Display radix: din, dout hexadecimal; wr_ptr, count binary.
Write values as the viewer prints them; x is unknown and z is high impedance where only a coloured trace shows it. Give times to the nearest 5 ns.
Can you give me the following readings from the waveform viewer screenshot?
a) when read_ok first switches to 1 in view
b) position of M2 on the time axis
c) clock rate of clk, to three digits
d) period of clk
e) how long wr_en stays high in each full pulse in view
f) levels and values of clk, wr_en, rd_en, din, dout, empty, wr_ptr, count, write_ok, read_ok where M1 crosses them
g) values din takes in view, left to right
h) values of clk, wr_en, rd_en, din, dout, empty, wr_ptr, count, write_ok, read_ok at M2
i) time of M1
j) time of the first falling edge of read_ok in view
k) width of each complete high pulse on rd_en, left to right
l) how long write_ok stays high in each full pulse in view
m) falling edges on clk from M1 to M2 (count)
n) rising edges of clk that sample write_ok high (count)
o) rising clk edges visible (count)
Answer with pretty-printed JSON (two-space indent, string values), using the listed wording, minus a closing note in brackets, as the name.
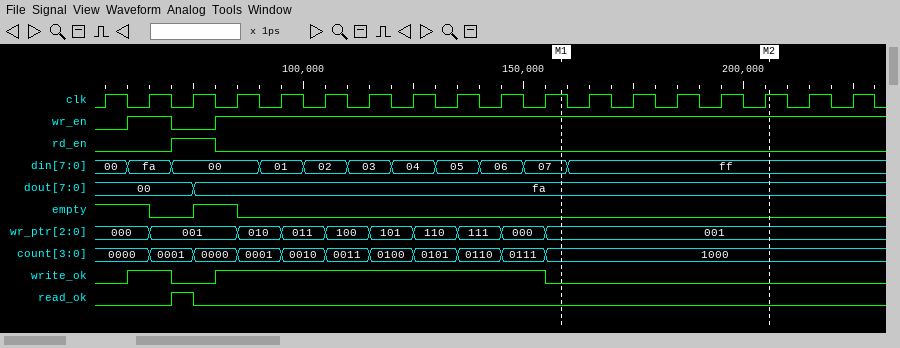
{
  "when read_ok first switches to 1 in view": "70 ns",
  "position of M2 on the time axis": "205 ns",
  "clock rate of clk, to three digits": "100 MHz",
  "period of clk": "10 ns",
  "how long wr_en stays high in each full pulse in view": "10 ns",
  "levels and values of clk, wr_en, rd_en, din, dout, empty, wr_ptr, count, write_ok, read_ok where M1 crosses them": "clk=1, wr_en=1, rd_en=0, din=07, dout=fa, empty=0, wr_ptr=001, count=1000, write_ok=0, read_ok=0",
  "values din takes in view, left to right": "00, fa, 00, 01, 02, 03, 04, 05, 06, 07, ff",
  "values of clk, wr_en, rd_en, din, dout, empty, wr_ptr, count, write_ok, read_ok at M2": "clk=1, wr_en=1, rd_en=0, din=ff, dout=fa, empty=0, wr_ptr=001, count=1000, write_ok=0, read_ok=0",
  "time of M1": "160 ns",
  "time of the first falling edge of read_ok in view": "75 ns",
  "width of each complete high pulse on rd_en, left to right": "10 ns",
  "how long write_ok stays high in each full pulse in view": "10 ns, 75 ns",
  "falling edges on clk from M1 to M2": "5",
  "rising edges of clk that sample write_ok high": "9",
  "rising clk edges visible": "18"
}
